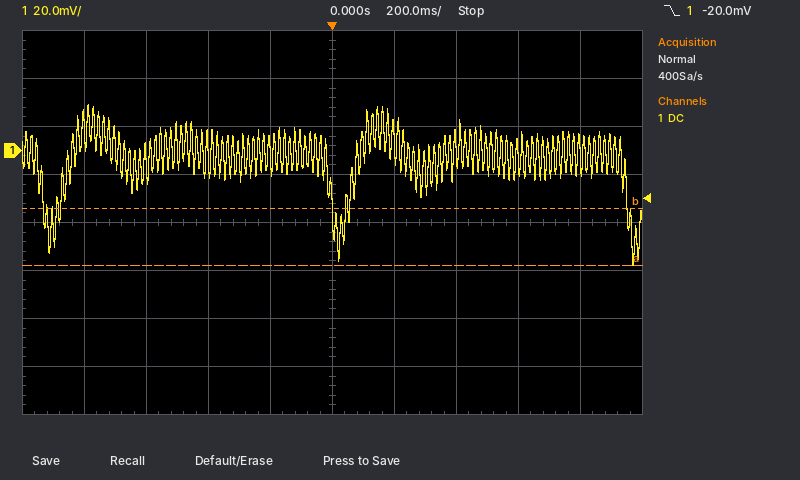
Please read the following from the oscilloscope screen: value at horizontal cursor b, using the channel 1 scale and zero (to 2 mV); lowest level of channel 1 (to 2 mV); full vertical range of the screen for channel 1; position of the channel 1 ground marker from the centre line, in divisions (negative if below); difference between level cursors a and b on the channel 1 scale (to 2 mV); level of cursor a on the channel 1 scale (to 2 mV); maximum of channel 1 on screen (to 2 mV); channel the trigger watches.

-24 mV
-48 mV
160 mV
+1.5 div
24 mV
-48 mV
20 mV
channel 1
